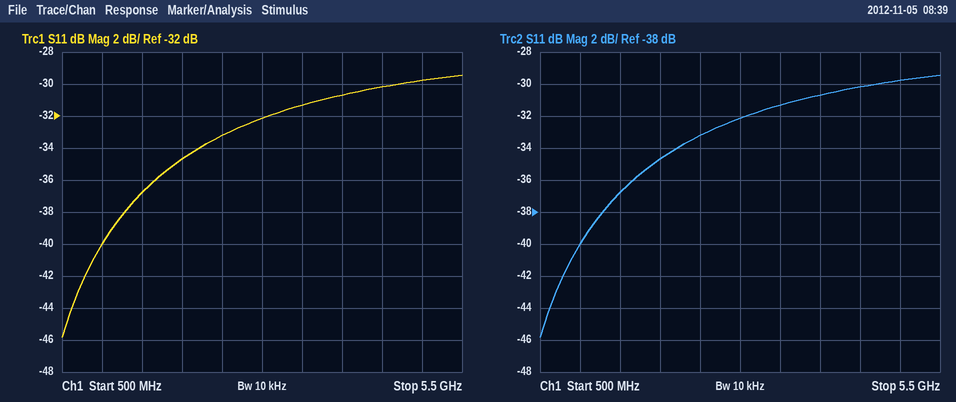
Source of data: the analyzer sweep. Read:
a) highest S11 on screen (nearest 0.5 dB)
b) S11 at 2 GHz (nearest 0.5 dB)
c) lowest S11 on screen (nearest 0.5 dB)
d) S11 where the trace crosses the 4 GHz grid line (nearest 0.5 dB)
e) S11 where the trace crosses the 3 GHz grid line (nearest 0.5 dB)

-29.5 dB
-34.5 dB
-46.0 dB
-30.5 dB
-32.0 dB
